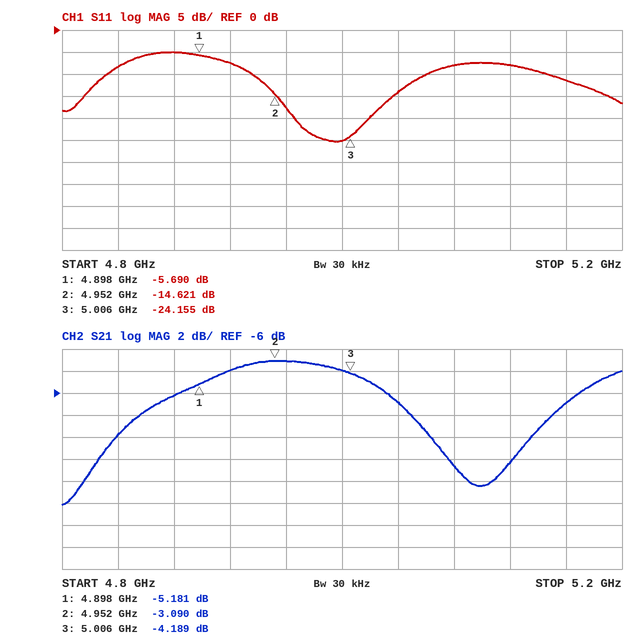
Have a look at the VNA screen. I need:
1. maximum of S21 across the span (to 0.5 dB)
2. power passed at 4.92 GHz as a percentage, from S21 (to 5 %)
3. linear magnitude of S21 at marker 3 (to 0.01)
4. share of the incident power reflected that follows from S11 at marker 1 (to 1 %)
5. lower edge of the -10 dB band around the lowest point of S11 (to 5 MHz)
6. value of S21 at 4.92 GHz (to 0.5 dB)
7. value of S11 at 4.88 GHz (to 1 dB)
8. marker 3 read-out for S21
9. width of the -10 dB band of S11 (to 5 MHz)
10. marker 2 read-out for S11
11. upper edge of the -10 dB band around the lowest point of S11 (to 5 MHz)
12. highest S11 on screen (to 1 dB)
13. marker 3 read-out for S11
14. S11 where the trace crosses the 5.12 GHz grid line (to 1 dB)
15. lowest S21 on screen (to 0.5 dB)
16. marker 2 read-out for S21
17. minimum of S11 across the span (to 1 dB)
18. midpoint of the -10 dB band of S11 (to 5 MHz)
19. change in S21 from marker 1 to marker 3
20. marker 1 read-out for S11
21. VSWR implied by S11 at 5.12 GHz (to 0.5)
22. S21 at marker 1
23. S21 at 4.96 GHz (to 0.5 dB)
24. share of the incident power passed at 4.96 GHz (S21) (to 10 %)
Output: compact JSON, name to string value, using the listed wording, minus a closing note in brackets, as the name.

{"maximum of S21 across the span": "-3.0 dB", "power passed at 4.92 GHz as a percentage, from S21": "40 %", "linear magnitude of S21 at marker 3": "0.62", "share of the incident power reflected that follows from S11 at marker 1": "27 %", "lower edge of the -10 dB band around the lowest point of S11": "4.935 GHz", "value of S21 at 4.92 GHz": "-4.0 dB", "value of S11 at 4.88 GHz": "-5 dB", "marker 3 read-out for S21": "-4.189 dB", "width of the -10 dB band of S11": "125 MHz", "marker 2 read-out for S11": "-14.621 dB", "upper edge of the -10 dB band around the lowest point of S11": "5.060 GHz", "highest S11 on screen": "-5 dB", "marker 3 read-out for S11": "-24.155 dB", "S11 where the trace crosses the 5.12 GHz grid line": "-8 dB", "lowest S21 on screen": "-16.0 dB", "marker 2 read-out for S21": "-3.090 dB", "minimum of S11 across the span": "-25 dB", "midpoint of the -10 dB band of S11": "5.000 GHz", "change in S21 from marker 1 to marker 3": "0.992 dB", "marker 1 read-out for S11": "-5.690 dB", "VSWR implied by S11 at 5.12 GHz": "2.5", "S21 at marker 1": "-5.181 dB", "S21 at 4.96 GHz": "-3.0 dB", "share of the incident power passed at 4.96 GHz (S21)": "50 %"}
